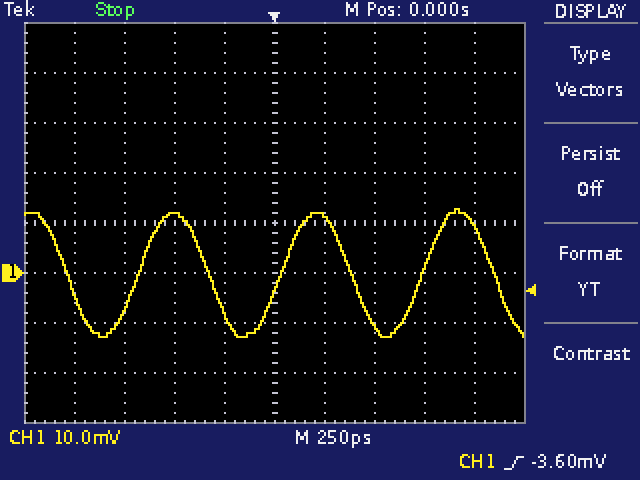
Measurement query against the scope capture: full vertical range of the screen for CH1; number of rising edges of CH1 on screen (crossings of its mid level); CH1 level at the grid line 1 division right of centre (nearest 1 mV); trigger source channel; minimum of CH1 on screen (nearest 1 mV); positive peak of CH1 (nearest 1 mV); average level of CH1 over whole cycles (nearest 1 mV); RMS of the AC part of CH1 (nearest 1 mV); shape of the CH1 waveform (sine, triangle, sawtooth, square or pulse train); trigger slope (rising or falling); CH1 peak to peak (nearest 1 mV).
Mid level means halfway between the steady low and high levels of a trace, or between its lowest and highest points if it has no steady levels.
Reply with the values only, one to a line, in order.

80 mV
3
11 mV
CH1
-13 mV
13 mV
0 mV
9 mV
sine
rising
26 mV
